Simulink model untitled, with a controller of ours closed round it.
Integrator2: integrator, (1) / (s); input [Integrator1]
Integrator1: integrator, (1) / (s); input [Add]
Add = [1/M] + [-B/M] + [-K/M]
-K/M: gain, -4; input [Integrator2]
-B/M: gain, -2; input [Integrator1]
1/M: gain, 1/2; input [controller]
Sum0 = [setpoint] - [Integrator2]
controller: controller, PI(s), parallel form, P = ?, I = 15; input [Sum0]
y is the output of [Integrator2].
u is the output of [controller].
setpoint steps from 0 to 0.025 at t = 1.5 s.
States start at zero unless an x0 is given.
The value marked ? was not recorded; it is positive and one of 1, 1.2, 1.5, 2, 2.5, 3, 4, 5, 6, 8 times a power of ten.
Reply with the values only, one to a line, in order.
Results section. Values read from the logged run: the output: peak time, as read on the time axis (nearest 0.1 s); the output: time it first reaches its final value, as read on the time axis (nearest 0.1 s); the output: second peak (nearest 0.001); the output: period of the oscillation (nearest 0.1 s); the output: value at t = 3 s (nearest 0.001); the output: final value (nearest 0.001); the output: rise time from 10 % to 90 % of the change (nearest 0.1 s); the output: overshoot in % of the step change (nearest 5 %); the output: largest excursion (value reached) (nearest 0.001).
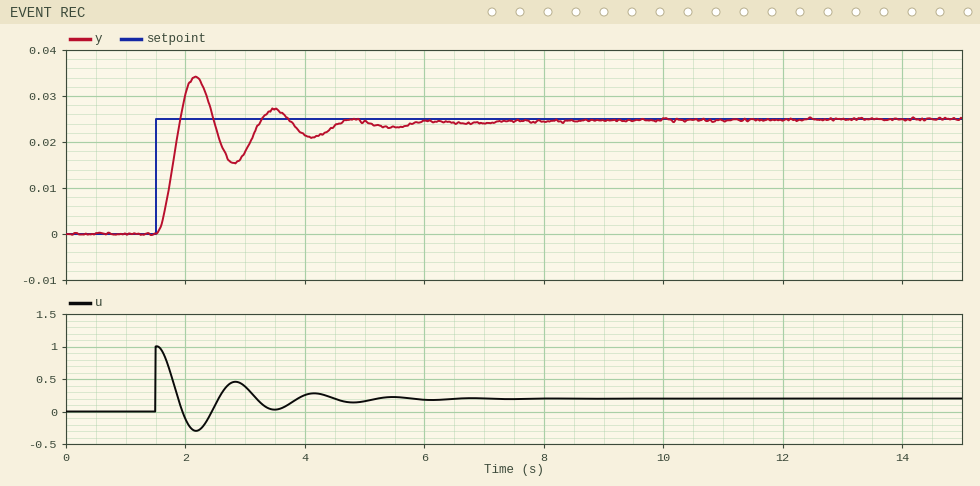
2.2 s
1.9 s
0.027
1.3 s
0.018
0.025
0.3 s
35 %
0.034
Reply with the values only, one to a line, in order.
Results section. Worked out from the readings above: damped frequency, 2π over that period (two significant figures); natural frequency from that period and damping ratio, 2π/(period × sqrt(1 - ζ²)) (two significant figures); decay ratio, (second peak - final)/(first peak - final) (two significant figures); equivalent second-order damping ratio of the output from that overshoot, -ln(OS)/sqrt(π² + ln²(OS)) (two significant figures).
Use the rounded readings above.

4.8 rad/s
5.1 rad/s
0.22
0.32
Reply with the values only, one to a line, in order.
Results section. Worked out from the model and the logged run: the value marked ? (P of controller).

40
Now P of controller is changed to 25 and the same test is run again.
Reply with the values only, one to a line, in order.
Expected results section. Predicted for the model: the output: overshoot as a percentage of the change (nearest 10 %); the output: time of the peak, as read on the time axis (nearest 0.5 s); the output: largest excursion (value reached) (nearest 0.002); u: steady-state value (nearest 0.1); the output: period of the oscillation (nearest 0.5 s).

30 %
2.5 s
0.032
0.2
1.5 s
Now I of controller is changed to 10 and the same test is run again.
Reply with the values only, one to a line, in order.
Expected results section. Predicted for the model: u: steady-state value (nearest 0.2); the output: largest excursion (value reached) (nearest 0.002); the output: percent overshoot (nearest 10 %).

0.2
0.034
30 %
